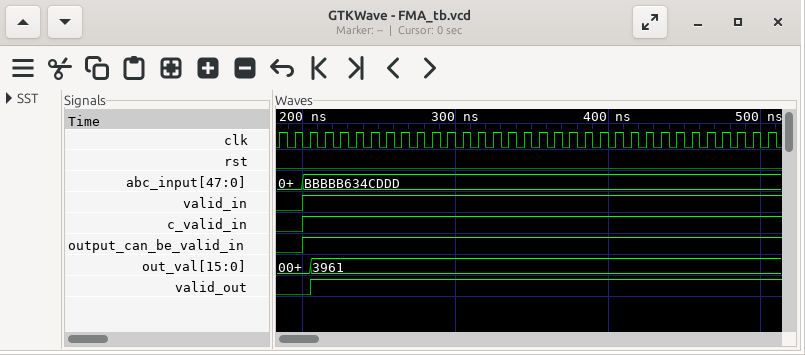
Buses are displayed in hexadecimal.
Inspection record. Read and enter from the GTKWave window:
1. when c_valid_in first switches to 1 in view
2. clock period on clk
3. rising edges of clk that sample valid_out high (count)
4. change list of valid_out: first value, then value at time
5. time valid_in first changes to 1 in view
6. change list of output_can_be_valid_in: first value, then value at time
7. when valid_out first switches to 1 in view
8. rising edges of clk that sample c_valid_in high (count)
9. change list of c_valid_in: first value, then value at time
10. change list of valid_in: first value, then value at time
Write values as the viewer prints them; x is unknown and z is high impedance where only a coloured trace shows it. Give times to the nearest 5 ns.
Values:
200 ns
10 ns
30
0, 1 at 205 ns
200 ns
0, 1 at 200 ns
205 ns
31
0, 1 at 200 ns
0, 1 at 200 ns
